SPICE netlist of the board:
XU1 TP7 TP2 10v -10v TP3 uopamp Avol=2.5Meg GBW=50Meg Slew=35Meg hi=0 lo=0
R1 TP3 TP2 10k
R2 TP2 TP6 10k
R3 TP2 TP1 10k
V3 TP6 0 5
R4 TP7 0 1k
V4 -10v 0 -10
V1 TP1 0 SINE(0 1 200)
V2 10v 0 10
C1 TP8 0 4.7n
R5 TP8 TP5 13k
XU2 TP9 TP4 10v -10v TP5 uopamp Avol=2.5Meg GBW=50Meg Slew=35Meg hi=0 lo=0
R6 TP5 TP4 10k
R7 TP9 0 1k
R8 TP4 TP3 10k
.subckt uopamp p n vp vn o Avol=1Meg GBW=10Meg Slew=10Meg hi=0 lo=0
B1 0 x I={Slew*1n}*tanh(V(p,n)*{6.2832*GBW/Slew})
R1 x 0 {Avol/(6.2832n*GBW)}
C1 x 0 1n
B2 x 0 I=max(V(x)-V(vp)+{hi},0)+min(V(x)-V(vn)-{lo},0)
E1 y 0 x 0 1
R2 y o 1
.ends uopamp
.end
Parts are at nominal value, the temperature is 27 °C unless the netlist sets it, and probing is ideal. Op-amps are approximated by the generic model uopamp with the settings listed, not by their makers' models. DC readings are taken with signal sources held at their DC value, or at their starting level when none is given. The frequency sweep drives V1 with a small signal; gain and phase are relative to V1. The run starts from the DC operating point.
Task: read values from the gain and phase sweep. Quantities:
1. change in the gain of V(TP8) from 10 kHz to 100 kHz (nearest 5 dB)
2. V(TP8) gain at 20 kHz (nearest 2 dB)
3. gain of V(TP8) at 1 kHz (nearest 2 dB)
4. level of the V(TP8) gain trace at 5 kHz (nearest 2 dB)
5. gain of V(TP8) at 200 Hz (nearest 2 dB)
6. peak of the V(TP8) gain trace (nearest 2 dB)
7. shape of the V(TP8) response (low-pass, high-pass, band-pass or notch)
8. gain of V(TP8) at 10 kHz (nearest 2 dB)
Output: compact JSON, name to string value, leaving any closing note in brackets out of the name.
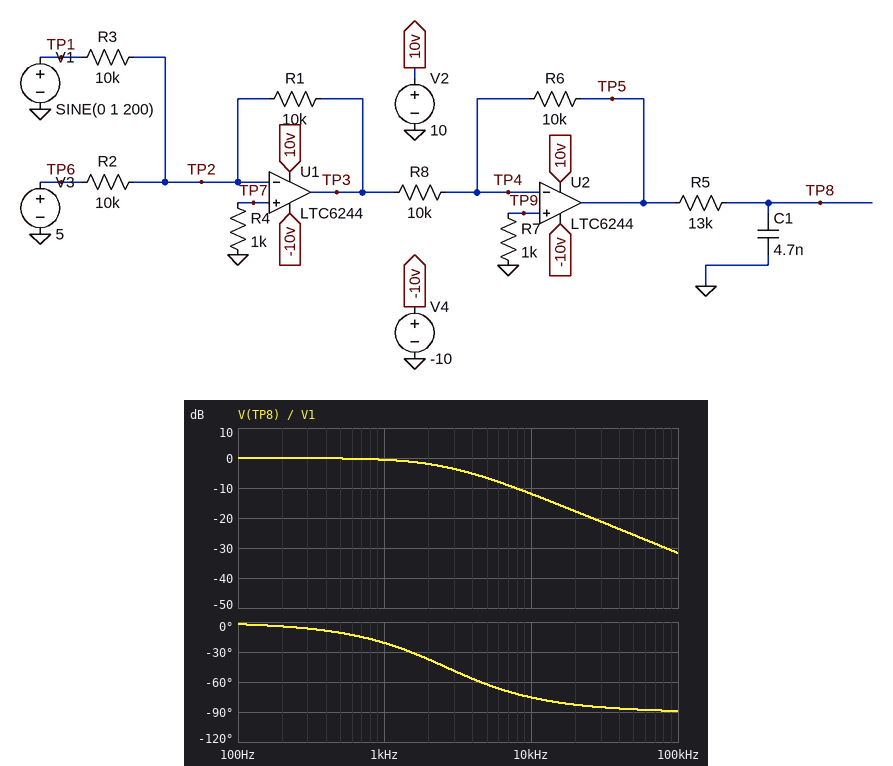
{"change in the gain of V(TP8) from 10 kHz to 100 kHz": "-20 dB", "V(TP8) gain at 20 kHz": "-18 dB", "gain of V(TP8) at 1 kHz": "0 dB", "level of the V(TP8) gain trace at 5 kHz": "-6 dB", "gain of V(TP8) at 200 Hz": "0 dB", "peak of the V(TP8) gain trace": "0 dB", "shape of the V(TP8) response": "low-pass", "gain of V(TP8) at 10 kHz": "-12 dB"}
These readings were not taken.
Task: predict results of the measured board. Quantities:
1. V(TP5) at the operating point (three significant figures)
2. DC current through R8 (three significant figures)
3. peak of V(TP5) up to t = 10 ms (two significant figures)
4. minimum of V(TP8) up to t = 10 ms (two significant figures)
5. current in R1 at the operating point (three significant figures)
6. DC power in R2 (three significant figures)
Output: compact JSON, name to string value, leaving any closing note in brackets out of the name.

{"V(TP5) at the operating point": "5.00 V", "DC current through R8": "500 µA", "peak of V(TP5) up to t = 10 ms": "6.0 V", "minimum of V(TP8) up to t = 10 ms": "4.0 V", "current in R1 at the operating point": "500 µA", "DC power in R2": "2.50 mW"}
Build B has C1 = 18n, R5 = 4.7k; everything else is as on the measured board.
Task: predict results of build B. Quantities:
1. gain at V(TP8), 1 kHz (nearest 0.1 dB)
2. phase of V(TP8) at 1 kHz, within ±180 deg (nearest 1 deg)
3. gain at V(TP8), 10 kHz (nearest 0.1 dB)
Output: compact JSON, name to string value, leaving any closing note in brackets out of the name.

{"gain at V(TP8), 1 kHz": "-1.1 dB", "phase of V(TP8) at 1 kHz, within ±180 deg": "-28 deg", "gain at V(TP8), 10 kHz": "-14.7 dB"}
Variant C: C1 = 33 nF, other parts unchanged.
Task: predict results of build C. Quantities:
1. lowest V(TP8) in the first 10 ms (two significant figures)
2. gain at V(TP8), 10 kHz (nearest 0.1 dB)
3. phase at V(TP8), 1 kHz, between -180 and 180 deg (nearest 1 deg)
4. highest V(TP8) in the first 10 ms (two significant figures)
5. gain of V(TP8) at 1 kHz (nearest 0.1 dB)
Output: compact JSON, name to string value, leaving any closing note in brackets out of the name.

{"lowest V(TP8) in the first 10 ms": "4.1 V", "gain at V(TP8), 10 kHz": "-28.6 dB", "phase at V(TP8), 1 kHz, between -180 and 180 deg": "-70 deg", "highest V(TP8) in the first 10 ms": "5.9 V", "gain of V(TP8) at 1 kHz": "-9.2 dB"}
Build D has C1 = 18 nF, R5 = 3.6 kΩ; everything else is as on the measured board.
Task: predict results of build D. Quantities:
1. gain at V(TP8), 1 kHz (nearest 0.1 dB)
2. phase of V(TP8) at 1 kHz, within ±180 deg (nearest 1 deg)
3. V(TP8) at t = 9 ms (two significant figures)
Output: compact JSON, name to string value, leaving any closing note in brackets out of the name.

{"gain at V(TP8), 1 kHz": "-0.7 dB", "phase of V(TP8) at 1 kHz, within ±180 deg": "-22 deg", "V(TP8) at t = 9 ms": "4.0 V"}
